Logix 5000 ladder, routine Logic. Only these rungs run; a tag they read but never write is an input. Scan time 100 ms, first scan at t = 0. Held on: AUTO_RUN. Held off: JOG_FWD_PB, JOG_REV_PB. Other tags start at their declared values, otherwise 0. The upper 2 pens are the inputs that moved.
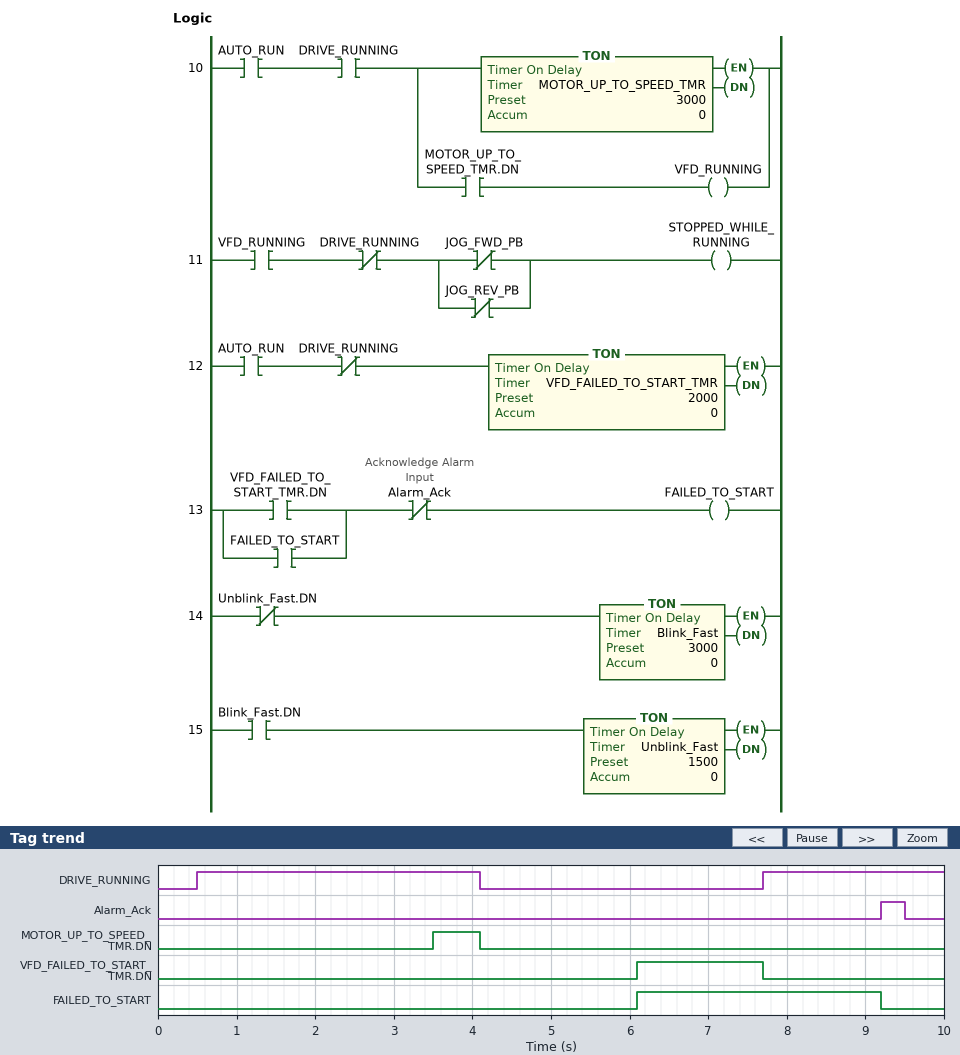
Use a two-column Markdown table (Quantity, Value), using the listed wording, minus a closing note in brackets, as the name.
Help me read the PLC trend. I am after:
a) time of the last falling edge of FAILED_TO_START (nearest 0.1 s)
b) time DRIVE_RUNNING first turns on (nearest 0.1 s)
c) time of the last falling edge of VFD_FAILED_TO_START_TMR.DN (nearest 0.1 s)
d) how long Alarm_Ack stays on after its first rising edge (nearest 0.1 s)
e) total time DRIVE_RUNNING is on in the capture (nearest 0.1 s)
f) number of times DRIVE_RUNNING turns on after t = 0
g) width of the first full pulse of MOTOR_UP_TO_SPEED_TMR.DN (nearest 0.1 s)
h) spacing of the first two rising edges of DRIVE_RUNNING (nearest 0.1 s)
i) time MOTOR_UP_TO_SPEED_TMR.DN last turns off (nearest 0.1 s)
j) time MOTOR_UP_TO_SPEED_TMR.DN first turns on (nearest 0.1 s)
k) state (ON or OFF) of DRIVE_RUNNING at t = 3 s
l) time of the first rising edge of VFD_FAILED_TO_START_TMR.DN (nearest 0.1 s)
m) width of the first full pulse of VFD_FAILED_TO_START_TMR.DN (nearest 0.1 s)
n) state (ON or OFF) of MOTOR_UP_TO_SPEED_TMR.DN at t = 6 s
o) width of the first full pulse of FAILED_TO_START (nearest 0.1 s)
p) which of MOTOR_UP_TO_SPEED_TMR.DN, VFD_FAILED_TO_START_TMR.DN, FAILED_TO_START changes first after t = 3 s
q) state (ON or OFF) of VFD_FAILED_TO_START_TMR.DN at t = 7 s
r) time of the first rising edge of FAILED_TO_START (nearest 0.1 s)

| Quantity | Value |
|---|---|
| time of the last falling edge of FAILED_TO_START | 9.2 s |
| time DRIVE_RUNNING first turns on | 0.5 s |
| time of the last falling edge of VFD_FAILED_TO_START_TMR.DN | 7.7 s |
| how long Alarm_Ack stays on after its first rising edge | 0.3 s |
| total time DRIVE_RUNNING is on in the capture | 5.9 s |
| number of times DRIVE_RUNNING turns on after t = 0 | 2 |
| width of the first full pulse of MOTOR_UP_TO_SPEED_TMR.DN | 0.6 s |
| spacing of the first two rising edges of DRIVE_RUNNING | 7.2 s |
| time MOTOR_UP_TO_SPEED_TMR.DN last turns off | 4.1 s |
| time MOTOR_UP_TO_SPEED_TMR.DN first turns on | 3.5 s |
| state (ON or OFF) of DRIVE_RUNNING at t = 3 s | ON |
| time of the first rising edge of VFD_FAILED_TO_START_TMR.DN | 6.1 s |
| width of the first full pulse of VFD_FAILED_TO_START_TMR.DN | 1.6 s |
| state (ON or OFF) of MOTOR_UP_TO_SPEED_TMR.DN at t = 6 s | OFF |
| width of the first full pulse of FAILED_TO_START | 3.1 s |
| which of MOTOR_UP_TO_SPEED_TMR.DN, VFD_FAILED_TO_START_TMR.DN, FAILED_TO_START changes first after t = 3 s | MOTOR_UP_TO_SPEED_TMR.DN |
| state (ON or OFF) of VFD_FAILED_TO_START_TMR.DN at t = 7 s | ON |
| time of the first rising edge of FAILED_TO_START | 6.1 s |
